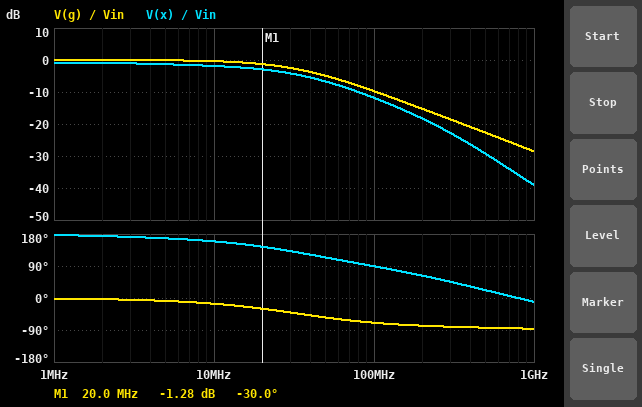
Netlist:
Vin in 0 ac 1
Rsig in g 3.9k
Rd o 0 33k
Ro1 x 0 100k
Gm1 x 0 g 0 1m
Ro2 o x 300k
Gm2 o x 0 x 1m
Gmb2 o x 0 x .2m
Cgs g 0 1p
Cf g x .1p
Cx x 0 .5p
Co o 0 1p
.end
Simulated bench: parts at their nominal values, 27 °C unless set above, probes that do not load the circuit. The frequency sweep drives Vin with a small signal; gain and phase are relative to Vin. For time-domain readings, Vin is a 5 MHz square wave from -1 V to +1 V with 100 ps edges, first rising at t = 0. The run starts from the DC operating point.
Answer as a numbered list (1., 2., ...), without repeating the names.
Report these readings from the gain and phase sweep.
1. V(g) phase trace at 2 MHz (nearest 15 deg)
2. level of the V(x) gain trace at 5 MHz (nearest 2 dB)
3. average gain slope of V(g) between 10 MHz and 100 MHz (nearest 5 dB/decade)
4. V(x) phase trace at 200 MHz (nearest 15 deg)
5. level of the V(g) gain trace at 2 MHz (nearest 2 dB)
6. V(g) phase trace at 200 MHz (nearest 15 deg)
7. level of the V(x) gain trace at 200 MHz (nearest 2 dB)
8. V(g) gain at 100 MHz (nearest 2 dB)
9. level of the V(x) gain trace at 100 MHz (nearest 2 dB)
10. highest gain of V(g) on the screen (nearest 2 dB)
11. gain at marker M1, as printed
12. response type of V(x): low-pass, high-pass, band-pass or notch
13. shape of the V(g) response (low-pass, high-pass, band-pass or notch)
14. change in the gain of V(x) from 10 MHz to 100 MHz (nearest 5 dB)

1. 0 deg
2. -2 dB
3. -10 dB/decade
4. 60 deg
5. 0 dB
6. -75 deg
7. -18 dB
8. -10 dB
9. -12 dB
10. 0 dB
11. -1.28 dB
12. low-pass
13. low-pass
14. -10 dB
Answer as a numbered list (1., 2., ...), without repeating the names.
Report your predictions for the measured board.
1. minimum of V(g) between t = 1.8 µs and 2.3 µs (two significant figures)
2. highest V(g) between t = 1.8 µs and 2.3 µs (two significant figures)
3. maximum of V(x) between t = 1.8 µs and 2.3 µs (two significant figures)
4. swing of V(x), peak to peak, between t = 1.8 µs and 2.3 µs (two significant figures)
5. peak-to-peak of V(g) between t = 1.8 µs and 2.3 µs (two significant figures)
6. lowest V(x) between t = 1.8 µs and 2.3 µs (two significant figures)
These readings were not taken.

1. -1.0 V
2. 1.0 V
3. 910 mV
4. 1.8 V
5. 2.0 V
6. -910 mV
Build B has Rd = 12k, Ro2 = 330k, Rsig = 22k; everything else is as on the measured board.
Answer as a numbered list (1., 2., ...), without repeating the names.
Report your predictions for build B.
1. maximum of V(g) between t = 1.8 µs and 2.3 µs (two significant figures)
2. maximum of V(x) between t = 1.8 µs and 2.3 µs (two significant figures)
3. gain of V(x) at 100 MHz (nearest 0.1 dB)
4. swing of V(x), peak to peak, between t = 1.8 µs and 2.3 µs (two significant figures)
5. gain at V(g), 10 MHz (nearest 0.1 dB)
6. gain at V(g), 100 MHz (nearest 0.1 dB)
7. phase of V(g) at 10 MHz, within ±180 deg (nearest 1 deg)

1. 960 mV
2. 820 mV
3. -26.3 dB
4. 1.6 V
5. -5.7 dB
6. -24.2 dB
7. -58 deg
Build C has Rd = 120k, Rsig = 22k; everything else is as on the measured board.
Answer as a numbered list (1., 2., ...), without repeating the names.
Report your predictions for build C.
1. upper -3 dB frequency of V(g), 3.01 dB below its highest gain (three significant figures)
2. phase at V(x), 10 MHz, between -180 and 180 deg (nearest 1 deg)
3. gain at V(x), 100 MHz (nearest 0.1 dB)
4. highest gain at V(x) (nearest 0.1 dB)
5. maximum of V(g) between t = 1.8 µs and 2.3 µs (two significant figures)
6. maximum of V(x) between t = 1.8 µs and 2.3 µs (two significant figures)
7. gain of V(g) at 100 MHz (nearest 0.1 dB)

1. 6.07 MHz
2. 117 deg
3. -26.3 dB
4. 1.2 dB
5. 950 mV
6. 860 mV
7. -24.2 dB
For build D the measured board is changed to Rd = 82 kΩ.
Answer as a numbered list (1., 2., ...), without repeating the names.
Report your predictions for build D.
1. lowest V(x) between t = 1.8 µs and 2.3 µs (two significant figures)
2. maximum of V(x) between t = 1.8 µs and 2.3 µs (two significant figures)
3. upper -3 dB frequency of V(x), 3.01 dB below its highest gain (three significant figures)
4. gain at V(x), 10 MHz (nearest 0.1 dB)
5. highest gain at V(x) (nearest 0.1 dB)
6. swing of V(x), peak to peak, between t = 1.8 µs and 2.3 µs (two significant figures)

1. -940 mV
2. 940 mV
3. 16.8 MHz
4. -2.0 dB
5. 0.4 dB
6. 1.9 V
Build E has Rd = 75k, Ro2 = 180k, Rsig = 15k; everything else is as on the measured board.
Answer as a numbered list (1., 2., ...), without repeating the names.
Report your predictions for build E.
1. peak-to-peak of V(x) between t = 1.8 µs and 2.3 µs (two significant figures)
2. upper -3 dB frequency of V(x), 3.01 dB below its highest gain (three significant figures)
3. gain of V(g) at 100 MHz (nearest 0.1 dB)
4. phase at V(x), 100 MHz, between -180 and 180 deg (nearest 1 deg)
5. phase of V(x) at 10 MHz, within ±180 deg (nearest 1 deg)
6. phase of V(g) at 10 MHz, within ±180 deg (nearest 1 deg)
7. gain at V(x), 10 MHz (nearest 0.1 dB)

1. 1.9 V
2. 4.03 MHz
3. -20.9 dB
4. 75 deg
5. 125 deg
6. -48 deg
7. -5.1 dB
